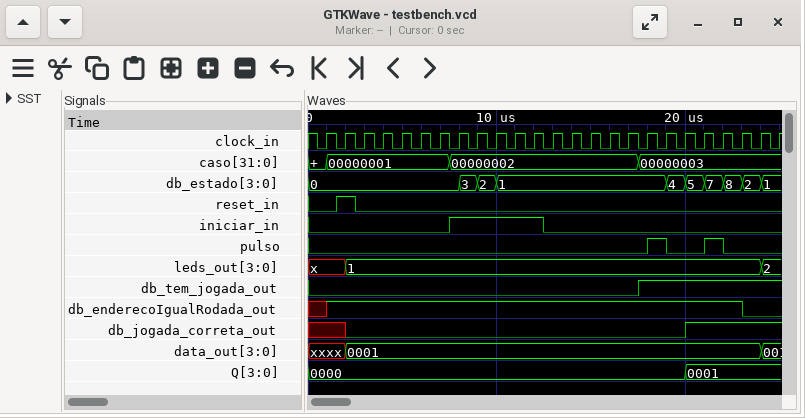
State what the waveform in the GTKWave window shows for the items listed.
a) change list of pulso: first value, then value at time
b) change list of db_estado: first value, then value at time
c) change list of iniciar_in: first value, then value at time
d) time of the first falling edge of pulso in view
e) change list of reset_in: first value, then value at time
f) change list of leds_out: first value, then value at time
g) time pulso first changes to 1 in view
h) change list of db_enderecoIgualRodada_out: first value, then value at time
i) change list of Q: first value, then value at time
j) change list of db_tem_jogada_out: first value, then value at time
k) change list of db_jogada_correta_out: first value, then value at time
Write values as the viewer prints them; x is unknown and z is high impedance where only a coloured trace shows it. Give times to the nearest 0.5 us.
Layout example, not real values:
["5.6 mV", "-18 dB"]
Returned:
["0, 1 at 18 us, 0 at 19 us, 1 at 21 us, 0 at 22 us", "0, 3 at 8 us, 2 at 9 us, 1 at 10 us, 4 at 19 us, 5 at 20 us, 7 at 21 us, 8 at 22 us, 2 at 23 us, 1 at 24 us", "0, 1 at 7.5 us, 0 at 12.5 us", "19 us", "0, 1 at 1.5 us, 0 at 2.5 us", "x, 1 at 2 us, 2 at 24 us", "18 us", "x, 1 at 1 us, 0 at 23 us", "0000, 0001 at 20 us", "0, 1 at 17.5 us", "x, 0 at 2 us, 1 at 20 us"]
